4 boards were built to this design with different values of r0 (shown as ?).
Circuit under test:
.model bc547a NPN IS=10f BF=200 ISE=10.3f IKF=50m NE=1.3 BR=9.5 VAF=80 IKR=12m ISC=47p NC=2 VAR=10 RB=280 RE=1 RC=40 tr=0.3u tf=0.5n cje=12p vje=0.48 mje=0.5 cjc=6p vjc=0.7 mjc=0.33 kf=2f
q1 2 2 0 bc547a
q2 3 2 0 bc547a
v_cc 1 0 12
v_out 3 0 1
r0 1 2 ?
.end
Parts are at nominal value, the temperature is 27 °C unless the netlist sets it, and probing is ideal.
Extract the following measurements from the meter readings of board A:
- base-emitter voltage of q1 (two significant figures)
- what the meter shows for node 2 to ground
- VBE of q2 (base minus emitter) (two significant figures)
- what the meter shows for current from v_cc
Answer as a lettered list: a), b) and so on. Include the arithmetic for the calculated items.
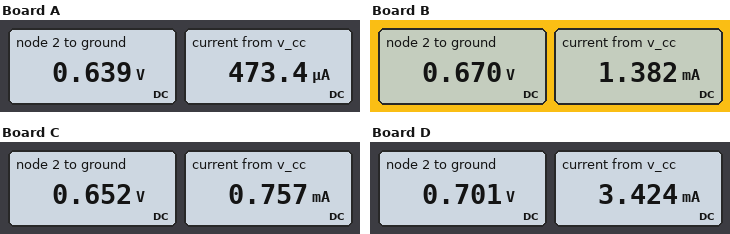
a) 639 mV = 640 mV
b) 0.639 V
c) 639 mV = 640 mV
d) 473.4 µA
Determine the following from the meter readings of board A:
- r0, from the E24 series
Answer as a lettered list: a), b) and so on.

a) 24 kΩ
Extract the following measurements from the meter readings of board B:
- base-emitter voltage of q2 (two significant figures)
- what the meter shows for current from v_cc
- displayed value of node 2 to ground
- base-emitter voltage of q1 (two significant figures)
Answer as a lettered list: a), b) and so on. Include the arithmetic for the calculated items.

a) 670 mV = 670 mV
b) 1.382 mA
c) 0.670 V
d) 670 mV = 670 mV
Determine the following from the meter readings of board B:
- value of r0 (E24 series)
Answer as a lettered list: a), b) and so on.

a) 8.2 kΩ
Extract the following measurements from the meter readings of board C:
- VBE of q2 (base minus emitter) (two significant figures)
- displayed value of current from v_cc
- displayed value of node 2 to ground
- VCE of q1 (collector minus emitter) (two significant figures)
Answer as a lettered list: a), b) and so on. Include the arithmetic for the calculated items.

a) 652 mV = 650 mV
b) 0.757 mA
c) 0.652 V
d) 652 mV = 650 mV
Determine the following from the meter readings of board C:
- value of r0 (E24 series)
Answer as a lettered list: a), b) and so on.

a) 15 kΩ
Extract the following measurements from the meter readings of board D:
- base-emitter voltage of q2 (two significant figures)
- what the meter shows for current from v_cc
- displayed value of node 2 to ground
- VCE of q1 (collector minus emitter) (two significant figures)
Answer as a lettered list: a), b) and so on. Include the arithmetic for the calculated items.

a) 701 mV = 700 mV
b) 3.424 mA
c) 0.701 V
d) 701 mV = 700 mV
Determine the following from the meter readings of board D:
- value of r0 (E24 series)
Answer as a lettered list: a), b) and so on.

a) 3.3 kΩ
